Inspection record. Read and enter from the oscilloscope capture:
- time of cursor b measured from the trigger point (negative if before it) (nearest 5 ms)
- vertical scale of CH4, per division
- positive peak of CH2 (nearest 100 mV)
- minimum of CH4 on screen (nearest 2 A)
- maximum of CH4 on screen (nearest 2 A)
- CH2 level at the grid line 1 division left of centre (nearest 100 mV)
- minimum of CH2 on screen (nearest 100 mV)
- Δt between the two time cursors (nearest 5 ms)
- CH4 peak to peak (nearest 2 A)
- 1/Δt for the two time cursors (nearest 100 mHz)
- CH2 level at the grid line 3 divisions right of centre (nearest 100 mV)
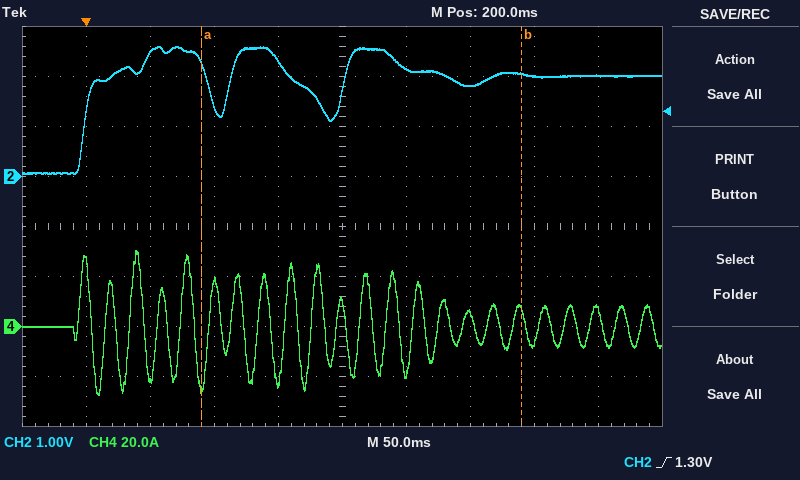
+340 ms
20 A
2.6 V
-28 A
30 A
2.3 V
100 mV
250 ms
58 A
4.0 Hz
2.0 V
